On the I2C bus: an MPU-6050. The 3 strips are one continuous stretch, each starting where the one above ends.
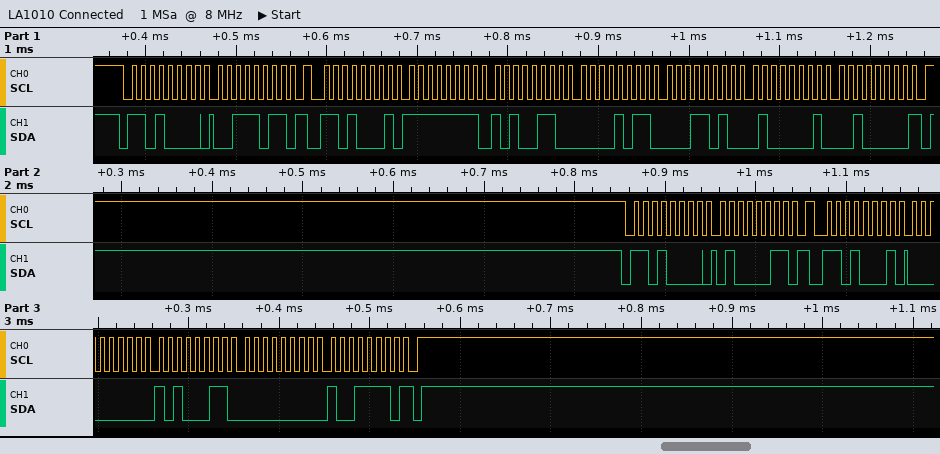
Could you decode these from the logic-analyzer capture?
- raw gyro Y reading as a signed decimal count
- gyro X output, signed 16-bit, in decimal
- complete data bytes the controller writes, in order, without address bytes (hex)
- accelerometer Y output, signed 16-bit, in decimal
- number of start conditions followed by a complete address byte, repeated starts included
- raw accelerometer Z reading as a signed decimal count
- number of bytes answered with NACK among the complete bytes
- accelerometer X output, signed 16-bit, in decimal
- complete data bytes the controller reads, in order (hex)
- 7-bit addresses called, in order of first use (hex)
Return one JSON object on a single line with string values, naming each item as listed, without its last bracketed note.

{"raw gyro Y reading as a signed decimal count": "158", "gyro X output, signed 16-bit, in decimal": "163", "complete data bytes the controller writes, in order, without address bytes": "3B 43", "accelerometer Y output, signed 16-bit, in decimal": "2842", "number of start conditions followed by a complete address byte, repeated starts included": "4", "raw accelerometer Z reading as a signed decimal count": "16672", "number of bytes answered with NACK among the complete bytes": "2", "accelerometer X output, signed 16-bit, in decimal": "-90", "complete data bytes the controller reads, in order": "FF A6 0B 1A 41 20 00 A3 00 9E", "7-bit addresses called, in order of first use": "0x68"}
